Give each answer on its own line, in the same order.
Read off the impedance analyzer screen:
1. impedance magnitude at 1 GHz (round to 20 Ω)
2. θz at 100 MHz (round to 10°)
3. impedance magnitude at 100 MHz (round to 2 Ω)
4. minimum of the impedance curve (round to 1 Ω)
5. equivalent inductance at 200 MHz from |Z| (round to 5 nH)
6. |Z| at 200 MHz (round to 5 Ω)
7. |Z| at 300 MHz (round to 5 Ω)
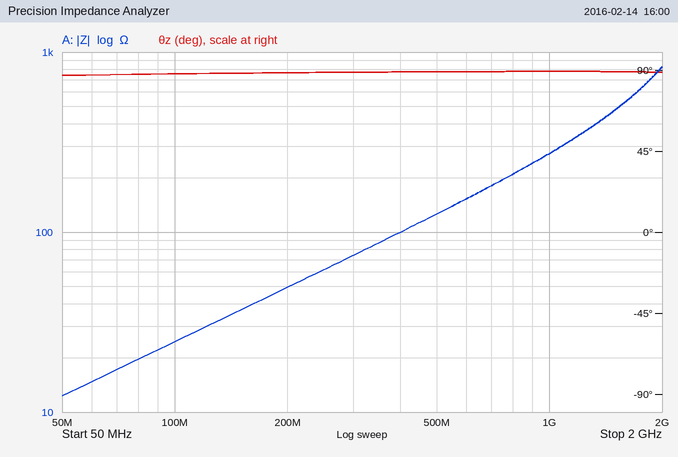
280 Ω
90°
24 Ω
12 Ω
40 nH
50 Ω
75 Ω
